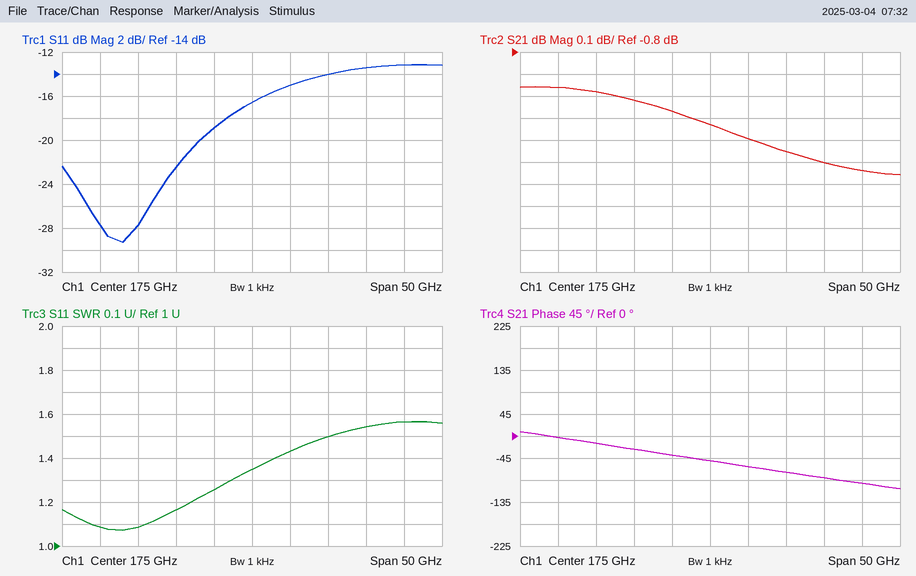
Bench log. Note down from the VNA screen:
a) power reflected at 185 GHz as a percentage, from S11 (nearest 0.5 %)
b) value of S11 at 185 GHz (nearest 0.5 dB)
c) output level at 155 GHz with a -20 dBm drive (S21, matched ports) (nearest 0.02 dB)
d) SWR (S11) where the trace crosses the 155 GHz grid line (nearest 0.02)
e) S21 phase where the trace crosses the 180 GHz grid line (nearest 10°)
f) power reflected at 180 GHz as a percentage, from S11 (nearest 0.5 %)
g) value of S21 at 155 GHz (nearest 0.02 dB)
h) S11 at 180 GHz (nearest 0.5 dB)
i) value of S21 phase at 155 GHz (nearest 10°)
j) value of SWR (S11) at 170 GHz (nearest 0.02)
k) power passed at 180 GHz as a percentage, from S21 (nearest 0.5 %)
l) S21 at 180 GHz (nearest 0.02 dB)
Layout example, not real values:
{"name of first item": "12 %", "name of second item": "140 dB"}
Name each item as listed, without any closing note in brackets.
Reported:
{"power reflected at 185 GHz as a percentage, from S11": "4.0 %", "value of S11 at 185 GHz": "-14.0 dB", "output level at 155 GHz with a -20 dBm drive (S21, matched ports)": "-20.96 dBm", "SWR (S11) where the trace crosses the 155 GHz grid line": "1.08", "S21 phase where the trace crosses the 180 GHz grid line": "-60°", "power reflected at 180 GHz as a percentage, from S11": "3.0 %", "value of S21 at 155 GHz": "-0.96 dB", "S11 at 180 GHz": "-15.0 dB", "value of S21 phase at 155 GHz": "0°", "value of SWR (S11) at 170 GHz": "1.26", "power passed at 180 GHz as a percentage, from S21": "76.0 %", "S21 at 180 GHz": "-1.20 dB"}
